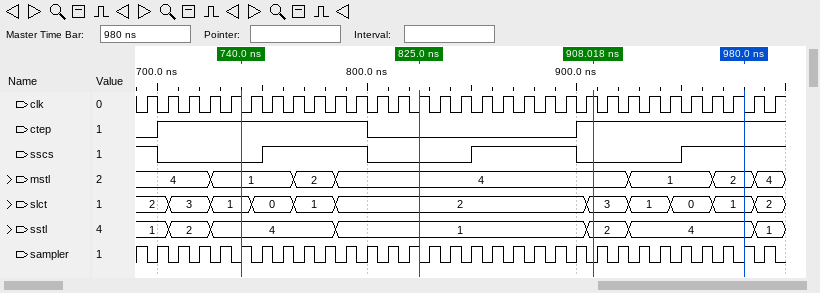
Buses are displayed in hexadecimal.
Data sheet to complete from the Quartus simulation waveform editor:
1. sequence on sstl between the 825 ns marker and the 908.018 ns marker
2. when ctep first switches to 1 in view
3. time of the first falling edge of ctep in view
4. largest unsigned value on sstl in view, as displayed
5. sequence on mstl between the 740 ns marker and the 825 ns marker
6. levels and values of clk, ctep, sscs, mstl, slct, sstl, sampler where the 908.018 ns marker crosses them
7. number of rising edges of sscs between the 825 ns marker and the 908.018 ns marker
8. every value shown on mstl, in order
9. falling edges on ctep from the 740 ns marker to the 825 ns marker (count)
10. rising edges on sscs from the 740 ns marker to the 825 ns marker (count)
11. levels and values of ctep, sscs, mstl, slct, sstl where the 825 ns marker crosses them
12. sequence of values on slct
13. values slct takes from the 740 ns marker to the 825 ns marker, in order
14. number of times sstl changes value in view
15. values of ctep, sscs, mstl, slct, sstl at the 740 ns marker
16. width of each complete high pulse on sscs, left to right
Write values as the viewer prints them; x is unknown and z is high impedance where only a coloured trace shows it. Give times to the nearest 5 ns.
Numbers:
1, 2
700 ns
800 ns
4
1, 2, 4
clk=1, ctep=1, sscs=0, mstl=4, slct=3, sstl=2, sampler=0
1
4, 1, 2, 4, 1, 2, 4
1
1
ctep=0, sscs=0, mstl=4, slct=2, sstl=1
2, 3, 1, 0, 1, 2, 3, 1, 0, 1, 2
1, 0, 1, 2
6
ctep=1, sscs=0, mstl=1, slct=1, sstl=4
50 ns, 50 ns
